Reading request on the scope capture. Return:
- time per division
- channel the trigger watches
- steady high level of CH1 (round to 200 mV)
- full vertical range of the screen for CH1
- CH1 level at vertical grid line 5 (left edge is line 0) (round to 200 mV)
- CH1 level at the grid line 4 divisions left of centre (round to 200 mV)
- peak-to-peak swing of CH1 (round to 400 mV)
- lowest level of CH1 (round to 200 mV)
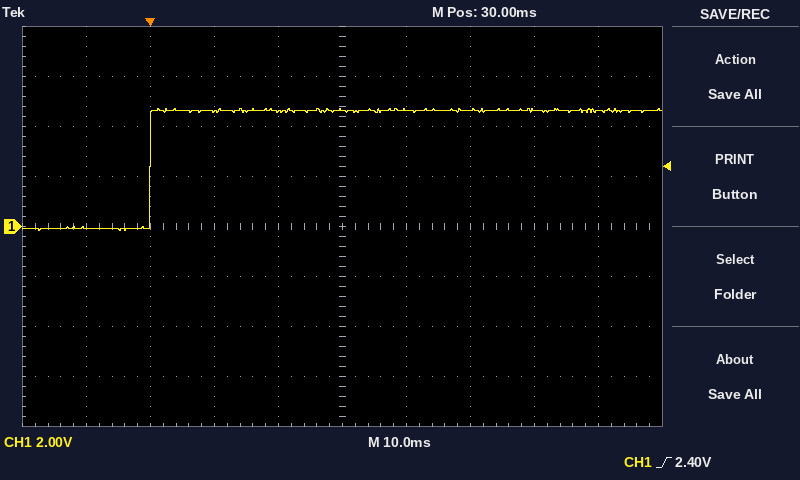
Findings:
10 ms
CH1
4.6 V
16 V
4.6 V
0.0 V
4.8 V
-200 mV
